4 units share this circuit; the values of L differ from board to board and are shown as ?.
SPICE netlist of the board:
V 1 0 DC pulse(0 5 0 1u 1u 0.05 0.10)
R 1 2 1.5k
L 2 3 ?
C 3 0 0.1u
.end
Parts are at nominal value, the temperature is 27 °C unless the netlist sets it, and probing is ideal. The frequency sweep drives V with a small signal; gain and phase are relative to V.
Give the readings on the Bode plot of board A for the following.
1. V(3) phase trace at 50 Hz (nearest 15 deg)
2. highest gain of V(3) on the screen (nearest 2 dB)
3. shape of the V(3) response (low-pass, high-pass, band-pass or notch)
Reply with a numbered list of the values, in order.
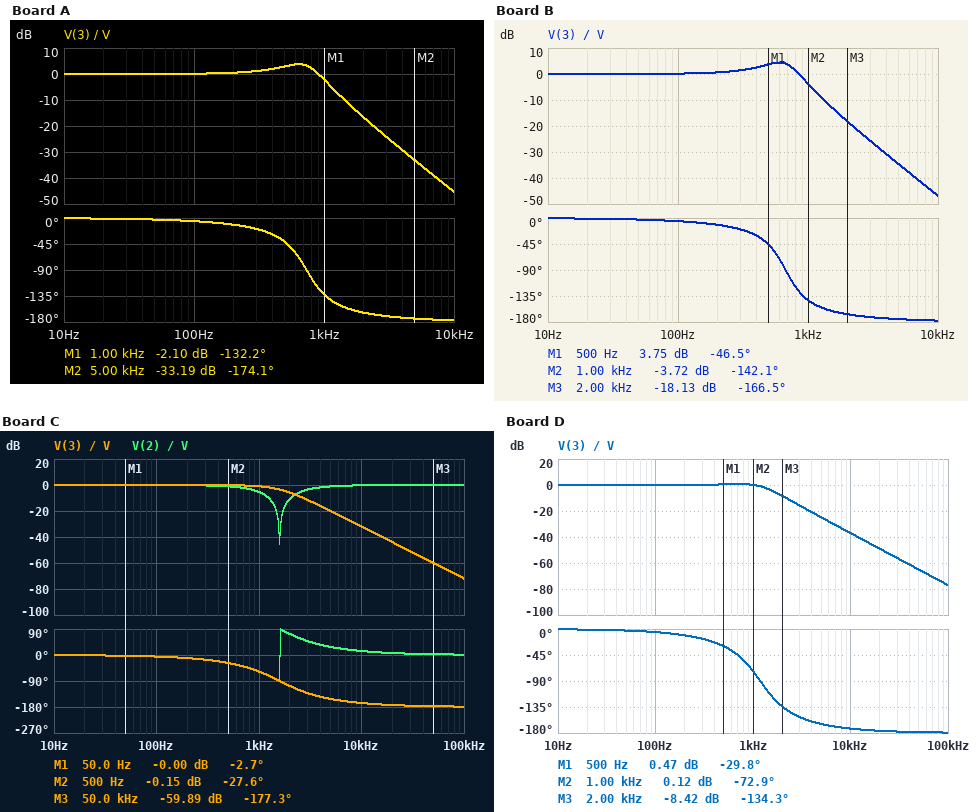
1. 0 deg
2. 4 dB
3. low-pass
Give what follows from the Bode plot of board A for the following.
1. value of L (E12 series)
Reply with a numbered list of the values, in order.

1. 470 mH
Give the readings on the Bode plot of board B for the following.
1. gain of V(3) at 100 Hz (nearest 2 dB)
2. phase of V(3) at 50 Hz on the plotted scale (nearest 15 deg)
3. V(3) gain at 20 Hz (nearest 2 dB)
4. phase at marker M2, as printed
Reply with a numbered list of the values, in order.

1. 0 dB
2. 0 deg
3. 0 dB
4. -142.1 deg
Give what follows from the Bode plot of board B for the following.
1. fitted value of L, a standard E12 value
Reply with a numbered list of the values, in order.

1. 560 mH
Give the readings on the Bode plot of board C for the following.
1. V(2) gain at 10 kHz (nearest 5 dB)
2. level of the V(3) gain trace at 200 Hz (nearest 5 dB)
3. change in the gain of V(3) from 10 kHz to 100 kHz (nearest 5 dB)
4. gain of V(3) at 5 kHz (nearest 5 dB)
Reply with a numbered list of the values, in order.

1. 0 dB
2. 0 dB
3. -40 dB
4. -20 dB
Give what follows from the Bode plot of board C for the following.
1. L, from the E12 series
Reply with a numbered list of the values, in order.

1. 100 mH
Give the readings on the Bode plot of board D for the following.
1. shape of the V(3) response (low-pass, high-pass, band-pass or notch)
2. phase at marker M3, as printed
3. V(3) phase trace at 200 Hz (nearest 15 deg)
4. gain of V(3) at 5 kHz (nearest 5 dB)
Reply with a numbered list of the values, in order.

1. low-pass
2. -134.3 deg
3. -15 deg
4. -25 dB
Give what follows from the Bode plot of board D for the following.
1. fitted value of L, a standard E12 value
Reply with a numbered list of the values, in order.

1. 180 mH
